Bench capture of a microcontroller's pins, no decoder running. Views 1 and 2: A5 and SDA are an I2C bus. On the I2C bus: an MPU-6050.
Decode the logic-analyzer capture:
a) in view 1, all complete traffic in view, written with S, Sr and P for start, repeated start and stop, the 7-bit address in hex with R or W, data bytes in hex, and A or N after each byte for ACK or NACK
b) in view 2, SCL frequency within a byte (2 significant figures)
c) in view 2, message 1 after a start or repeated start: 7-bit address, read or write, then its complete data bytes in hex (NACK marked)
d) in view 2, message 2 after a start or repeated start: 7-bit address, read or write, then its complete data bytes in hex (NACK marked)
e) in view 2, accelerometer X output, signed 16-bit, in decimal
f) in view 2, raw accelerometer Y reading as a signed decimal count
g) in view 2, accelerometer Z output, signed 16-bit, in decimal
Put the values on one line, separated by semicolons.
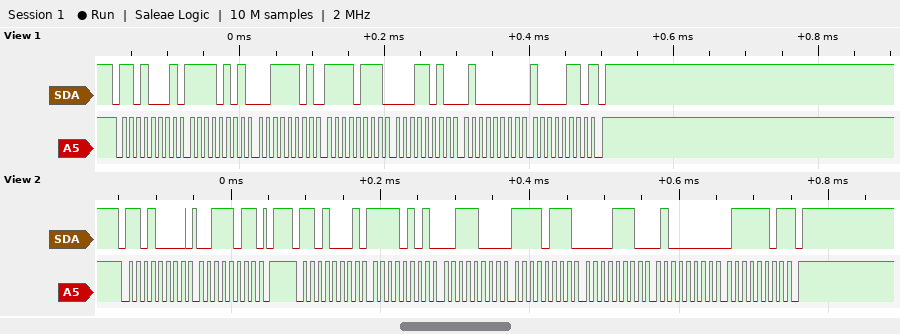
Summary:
S 68R A F5 A 3D A F7 A 1A A 40 A 86 N P; 100 kHz; 0x68 write: 3B; 0x68 read: F5 38 F7 0E 40 7D NACK; -2760; -2290; 16509
